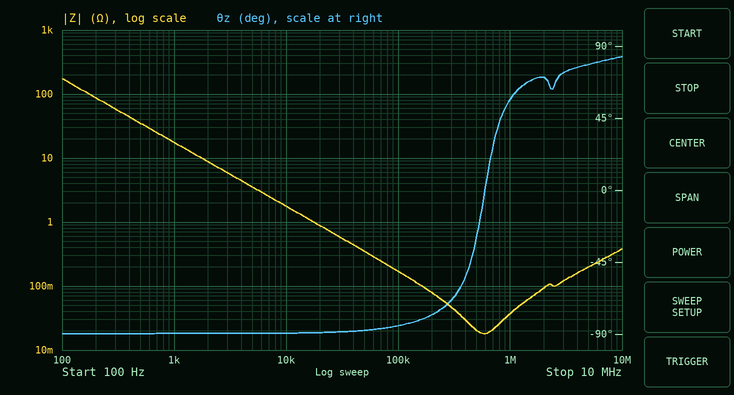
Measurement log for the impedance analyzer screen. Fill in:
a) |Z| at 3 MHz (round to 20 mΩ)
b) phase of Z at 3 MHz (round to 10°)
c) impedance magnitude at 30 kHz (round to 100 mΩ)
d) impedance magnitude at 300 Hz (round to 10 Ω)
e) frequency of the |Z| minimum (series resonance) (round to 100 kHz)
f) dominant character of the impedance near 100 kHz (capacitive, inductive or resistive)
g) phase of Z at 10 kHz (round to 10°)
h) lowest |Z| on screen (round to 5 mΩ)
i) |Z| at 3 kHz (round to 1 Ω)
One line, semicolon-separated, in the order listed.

120 mΩ; 70°; 600 mΩ; 60 Ω; 600 kHz; capacitive; -90°; 20 mΩ; 6 Ω
